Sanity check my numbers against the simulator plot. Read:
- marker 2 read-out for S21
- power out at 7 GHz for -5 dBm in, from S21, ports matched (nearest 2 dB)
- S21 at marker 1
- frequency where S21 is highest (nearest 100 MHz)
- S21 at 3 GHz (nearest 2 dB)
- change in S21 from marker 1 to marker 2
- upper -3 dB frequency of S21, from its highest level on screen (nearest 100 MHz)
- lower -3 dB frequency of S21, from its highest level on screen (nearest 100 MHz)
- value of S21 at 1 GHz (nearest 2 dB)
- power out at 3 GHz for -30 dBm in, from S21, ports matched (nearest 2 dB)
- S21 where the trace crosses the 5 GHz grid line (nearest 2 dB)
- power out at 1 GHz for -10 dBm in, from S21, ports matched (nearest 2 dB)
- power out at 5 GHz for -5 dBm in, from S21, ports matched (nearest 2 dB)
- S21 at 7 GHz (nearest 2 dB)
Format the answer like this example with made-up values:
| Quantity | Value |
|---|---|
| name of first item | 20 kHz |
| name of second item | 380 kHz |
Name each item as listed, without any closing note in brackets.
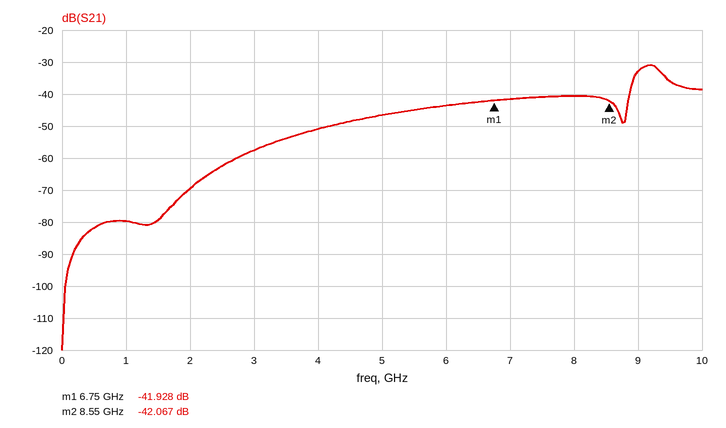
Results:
| Quantity | Value |
|---|---|
| marker 2 read-out for S21 | -42.067 dB |
| power out at 7 GHz for -5 dBm in, from S21, ports matched | -46 dBm |
| S21 at marker 1 | -41.928 dB |
| frequency where S21 is highest | 9.2 GHz |
| S21 at 3 GHz | -58 dB |
| change in S21 from marker 1 to marker 2 | -0.139 dB |
| upper -3 dB frequency of S21, from its highest level on screen | 9.4 GHz |
| lower -3 dB frequency of S21, from its highest level on screen | 9.0 GHz |
| value of S21 at 1 GHz | -80 dB |
| power out at 3 GHz for -30 dBm in, from S21, ports matched | -88 dBm |
| S21 where the trace crosses the 5 GHz grid line | -46 dB |
| power out at 1 GHz for -10 dBm in, from S21, ports matched | -90 dBm |
| power out at 5 GHz for -5 dBm in, from S21, ports matched | -52 dBm |
| S21 at 7 GHz | -42 dB |
